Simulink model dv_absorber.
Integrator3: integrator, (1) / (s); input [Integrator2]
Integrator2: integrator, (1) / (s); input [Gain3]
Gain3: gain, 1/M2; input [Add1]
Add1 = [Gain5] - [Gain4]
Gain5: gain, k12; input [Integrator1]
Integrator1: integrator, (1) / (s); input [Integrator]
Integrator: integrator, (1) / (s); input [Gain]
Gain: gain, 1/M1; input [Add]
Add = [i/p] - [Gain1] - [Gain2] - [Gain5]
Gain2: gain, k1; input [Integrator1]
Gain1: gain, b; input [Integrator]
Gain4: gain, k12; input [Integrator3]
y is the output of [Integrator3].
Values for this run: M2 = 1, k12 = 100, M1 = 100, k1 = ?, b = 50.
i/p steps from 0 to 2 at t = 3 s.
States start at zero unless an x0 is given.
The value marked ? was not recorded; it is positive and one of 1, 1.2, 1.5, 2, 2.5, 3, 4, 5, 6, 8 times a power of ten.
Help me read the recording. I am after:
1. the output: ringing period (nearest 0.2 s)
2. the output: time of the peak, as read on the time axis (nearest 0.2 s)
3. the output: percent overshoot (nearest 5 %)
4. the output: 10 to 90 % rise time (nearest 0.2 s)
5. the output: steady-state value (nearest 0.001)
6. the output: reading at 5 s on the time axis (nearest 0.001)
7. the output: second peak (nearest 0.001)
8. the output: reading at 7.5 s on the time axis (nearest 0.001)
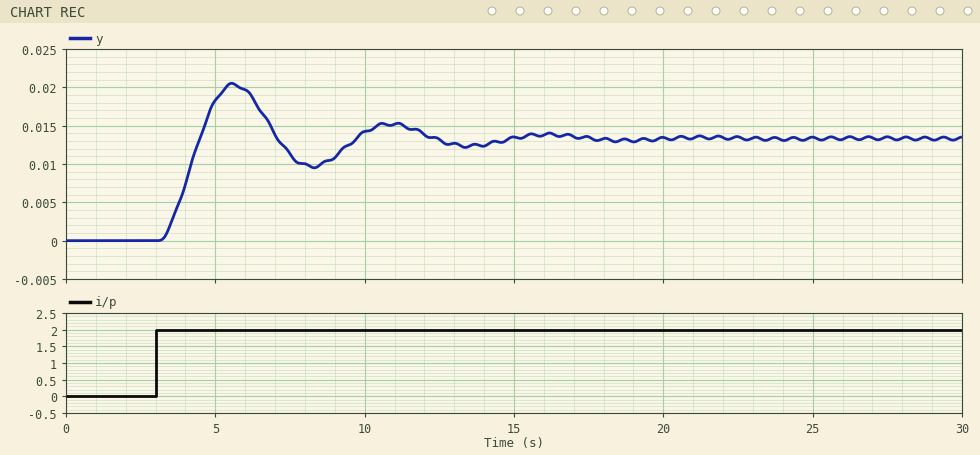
5.6 s
5.6 s
55 %
1.0 s
0.013
0.018
0.015
0.011
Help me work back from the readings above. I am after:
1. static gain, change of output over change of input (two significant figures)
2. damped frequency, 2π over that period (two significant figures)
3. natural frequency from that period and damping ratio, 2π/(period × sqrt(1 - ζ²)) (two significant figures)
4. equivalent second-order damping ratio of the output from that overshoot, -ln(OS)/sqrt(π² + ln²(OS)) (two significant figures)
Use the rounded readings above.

0.0065
1.1 rad/s
1.1 rad/s
0.19
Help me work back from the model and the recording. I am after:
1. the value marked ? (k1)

50
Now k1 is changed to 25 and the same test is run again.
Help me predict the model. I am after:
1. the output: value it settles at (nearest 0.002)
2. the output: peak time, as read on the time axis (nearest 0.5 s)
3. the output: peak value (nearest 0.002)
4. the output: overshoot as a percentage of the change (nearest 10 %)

0.016
6.0 s
0.024
50 %
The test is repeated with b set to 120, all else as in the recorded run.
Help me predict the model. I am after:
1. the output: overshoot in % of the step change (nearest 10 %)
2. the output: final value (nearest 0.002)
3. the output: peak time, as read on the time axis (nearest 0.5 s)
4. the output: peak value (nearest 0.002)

20 %
0.014
6.0 s
0.016
